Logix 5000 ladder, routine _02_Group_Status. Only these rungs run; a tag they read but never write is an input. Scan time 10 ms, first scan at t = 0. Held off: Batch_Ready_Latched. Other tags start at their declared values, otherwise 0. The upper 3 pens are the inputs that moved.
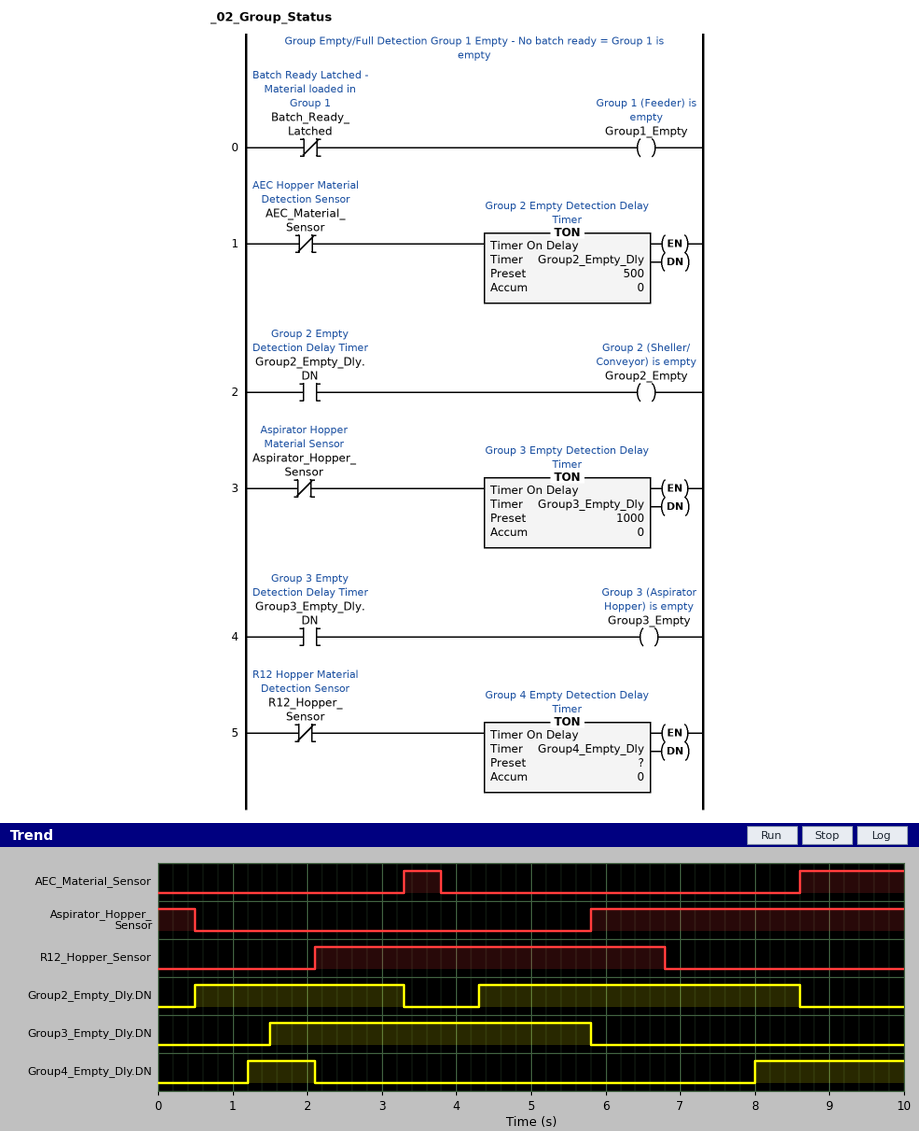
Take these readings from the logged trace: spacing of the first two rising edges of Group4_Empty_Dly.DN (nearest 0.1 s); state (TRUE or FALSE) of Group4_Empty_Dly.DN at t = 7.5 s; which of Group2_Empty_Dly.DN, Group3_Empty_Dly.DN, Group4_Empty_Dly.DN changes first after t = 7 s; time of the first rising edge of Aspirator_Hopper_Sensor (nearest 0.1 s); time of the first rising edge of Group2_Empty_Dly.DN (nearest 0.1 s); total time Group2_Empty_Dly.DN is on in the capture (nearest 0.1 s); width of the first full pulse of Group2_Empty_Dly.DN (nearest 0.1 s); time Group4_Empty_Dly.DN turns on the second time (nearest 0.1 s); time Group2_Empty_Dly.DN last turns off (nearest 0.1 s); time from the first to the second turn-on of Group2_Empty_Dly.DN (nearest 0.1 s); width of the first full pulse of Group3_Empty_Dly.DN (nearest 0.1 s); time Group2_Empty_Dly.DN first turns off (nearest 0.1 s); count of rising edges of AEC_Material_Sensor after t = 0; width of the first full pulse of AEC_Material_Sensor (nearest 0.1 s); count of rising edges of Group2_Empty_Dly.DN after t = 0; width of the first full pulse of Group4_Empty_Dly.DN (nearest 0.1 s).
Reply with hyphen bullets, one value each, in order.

- 6.8 s
- FALSE
- Group4_Empty_Dly.DN
- 5.8 s
- 0.5 s
- 7.1 s
- 2.8 s
- 8.0 s
- 8.6 s
- 3.8 s
- 4.3 s
- 3.3 s
- 2
- 0.5 s
- 2
- 0.9 s
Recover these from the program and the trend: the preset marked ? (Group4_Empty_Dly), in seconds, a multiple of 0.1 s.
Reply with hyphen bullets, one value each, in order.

- 1.2 s
